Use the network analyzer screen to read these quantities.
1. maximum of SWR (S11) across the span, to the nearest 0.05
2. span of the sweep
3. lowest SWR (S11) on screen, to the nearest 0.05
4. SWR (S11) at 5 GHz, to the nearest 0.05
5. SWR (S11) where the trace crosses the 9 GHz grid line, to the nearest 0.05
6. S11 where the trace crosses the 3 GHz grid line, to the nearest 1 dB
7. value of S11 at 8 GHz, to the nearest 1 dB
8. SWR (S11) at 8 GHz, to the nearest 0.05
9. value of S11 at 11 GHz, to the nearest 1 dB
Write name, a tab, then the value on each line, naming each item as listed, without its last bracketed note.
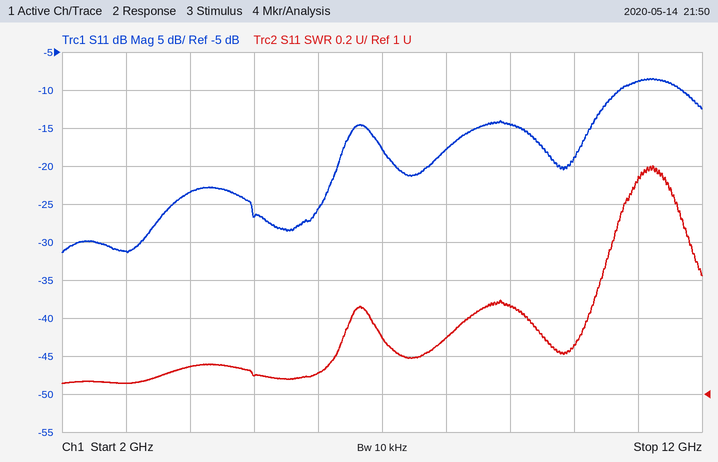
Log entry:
maximum of SWR (S11) across the span, to the nearest 0.05	2.20
span of the sweep	10 GHz
lowest SWR (S11) on screen, to the nearest 0.05	1.05
SWR (S11) at 5 GHz, to the nearest 0.05	1.10
SWR (S11) where the trace crosses the 9 GHz grid line, to the nearest 0.05	1.45
S11 where the trace crosses the 3 GHz grid line, to the nearest 1 dB	-31 dB
value of S11 at 8 GHz, to the nearest 1 dB	-18 dB
SWR (S11) at 8 GHz, to the nearest 0.05	1.30
value of S11 at 11 GHz, to the nearest 1 dB	-9 dB
